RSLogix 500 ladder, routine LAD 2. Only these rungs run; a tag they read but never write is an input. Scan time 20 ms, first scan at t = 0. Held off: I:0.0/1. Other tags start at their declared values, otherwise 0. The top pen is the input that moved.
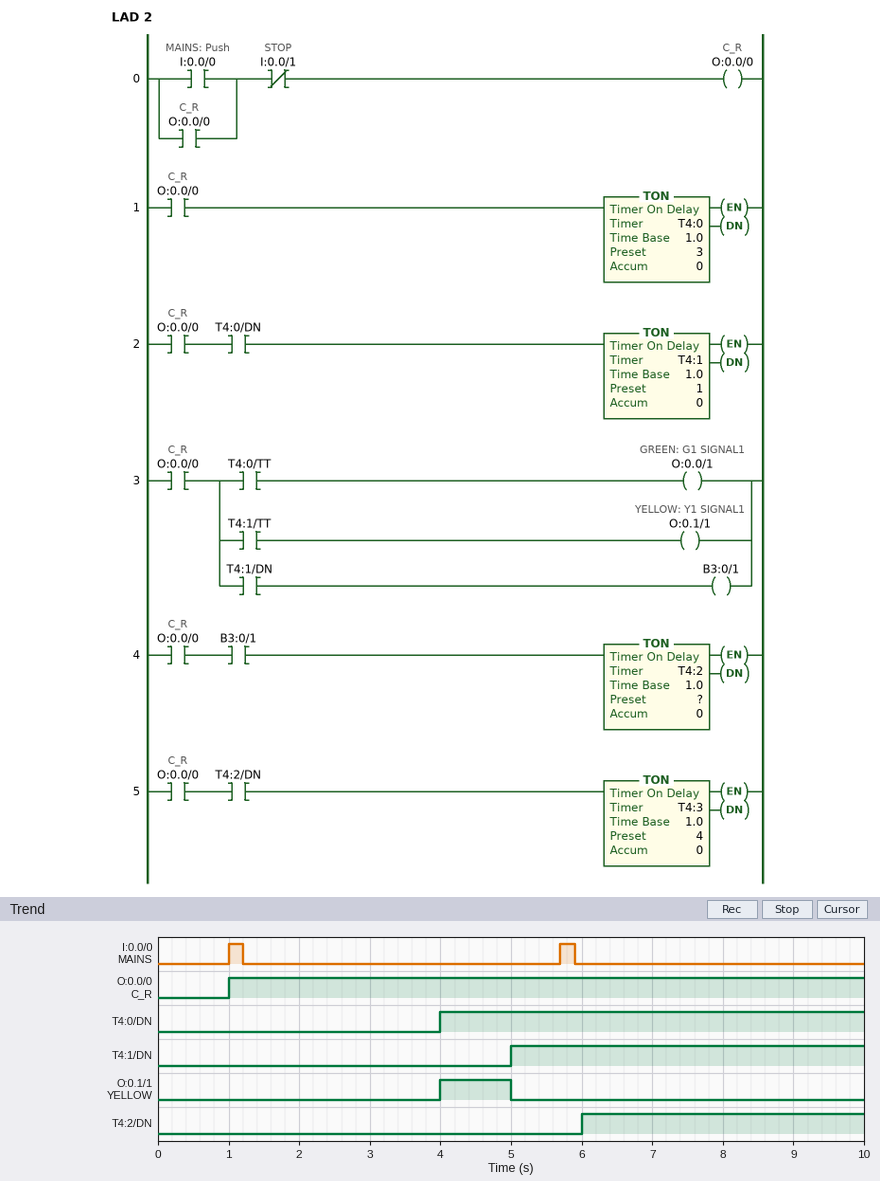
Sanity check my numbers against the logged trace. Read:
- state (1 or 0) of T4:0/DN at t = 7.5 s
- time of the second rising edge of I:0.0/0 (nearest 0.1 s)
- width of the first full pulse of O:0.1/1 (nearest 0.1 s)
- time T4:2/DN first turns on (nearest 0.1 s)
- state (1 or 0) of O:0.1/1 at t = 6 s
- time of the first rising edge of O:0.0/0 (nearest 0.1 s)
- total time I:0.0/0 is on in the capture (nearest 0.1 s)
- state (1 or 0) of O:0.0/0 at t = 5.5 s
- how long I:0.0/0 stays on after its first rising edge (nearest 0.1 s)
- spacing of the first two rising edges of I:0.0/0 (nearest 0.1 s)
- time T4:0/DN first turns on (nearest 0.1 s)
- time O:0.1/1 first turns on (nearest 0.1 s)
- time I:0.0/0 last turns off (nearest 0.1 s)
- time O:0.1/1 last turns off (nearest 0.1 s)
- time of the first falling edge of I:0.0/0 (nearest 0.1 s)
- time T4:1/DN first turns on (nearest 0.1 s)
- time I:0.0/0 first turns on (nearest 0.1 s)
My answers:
1
5.7 s
1.0 s
6.0 s
0
1.0 s
0.4 s
1
0.2 s
4.7 s
4.0 s
4.0 s
5.9 s
5.0 s
1.2 s
5.0 s
1.0 s
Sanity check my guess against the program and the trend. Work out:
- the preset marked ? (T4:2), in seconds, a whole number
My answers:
1 s
